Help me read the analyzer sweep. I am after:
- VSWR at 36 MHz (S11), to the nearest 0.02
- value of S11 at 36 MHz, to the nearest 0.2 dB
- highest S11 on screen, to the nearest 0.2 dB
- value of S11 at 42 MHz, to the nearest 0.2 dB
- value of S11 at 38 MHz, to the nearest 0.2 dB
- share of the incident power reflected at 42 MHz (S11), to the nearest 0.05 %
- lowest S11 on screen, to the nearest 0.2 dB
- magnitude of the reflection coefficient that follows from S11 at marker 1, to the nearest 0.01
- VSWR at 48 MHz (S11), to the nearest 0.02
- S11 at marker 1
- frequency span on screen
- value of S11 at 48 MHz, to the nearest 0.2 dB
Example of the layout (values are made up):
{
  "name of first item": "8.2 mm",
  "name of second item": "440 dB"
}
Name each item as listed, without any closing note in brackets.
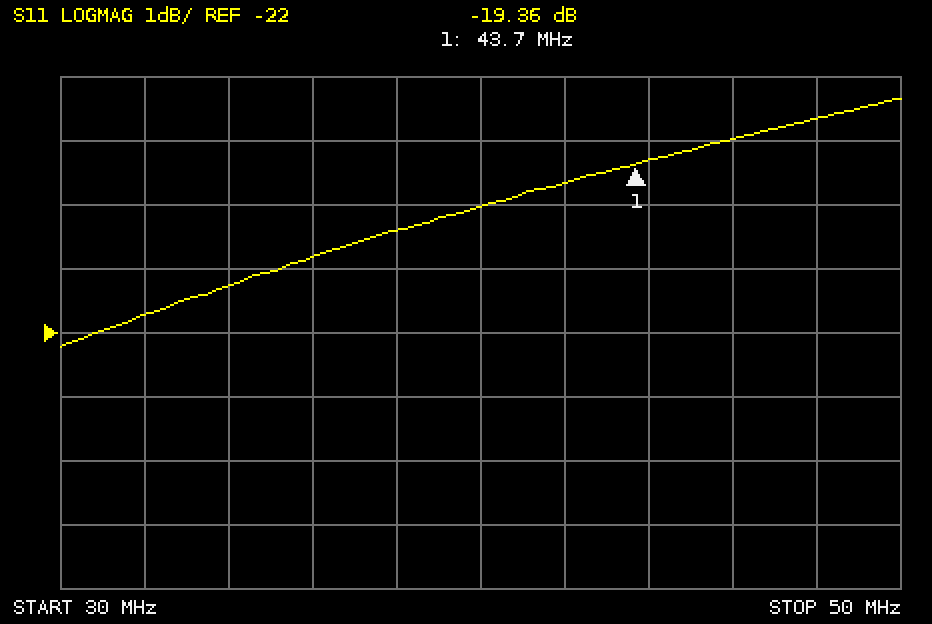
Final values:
{
  "VSWR at 36 MHz (S11), to the nearest 0.02": "1.20",
  "value of S11 at 36 MHz, to the nearest 0.2 dB": "-20.8 dB",
  "highest S11 on screen, to the nearest 0.2 dB": "-18.4 dB",
  "value of S11 at 42 MHz, to the nearest 0.2 dB": "-19.6 dB",
  "value of S11 at 38 MHz, to the nearest 0.2 dB": "-20.4 dB",
  "share of the incident power reflected at 42 MHz (S11), to the nearest 0.05 %": "1.10 %",
  "lowest S11 on screen, to the nearest 0.2 dB": "-22.2 dB",
  "magnitude of the reflection coefficient that follows from S11 at marker 1, to the nearest 0.01": "0.11",
  "VSWR at 48 MHz (S11), to the nearest 0.02": "1.26",
  "S11 at marker 1": "-19.36 dB",
  "frequency span on screen": "20 MHz",
  "value of S11 at 48 MHz, to the nearest 0.2 dB": "-18.6 dB"
}
